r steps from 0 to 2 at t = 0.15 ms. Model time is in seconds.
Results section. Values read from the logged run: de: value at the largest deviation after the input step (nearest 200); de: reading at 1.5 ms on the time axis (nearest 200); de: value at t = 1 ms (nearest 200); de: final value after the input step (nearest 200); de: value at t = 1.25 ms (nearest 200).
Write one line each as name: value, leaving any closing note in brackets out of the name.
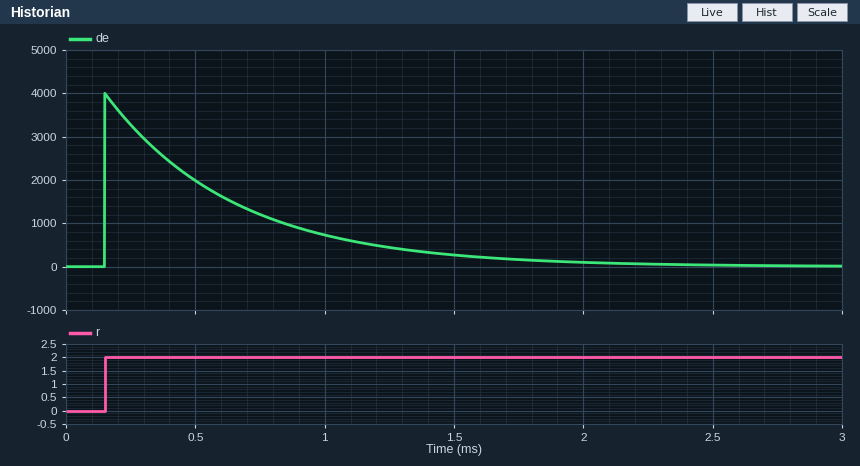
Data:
de: value at the largest deviation after the input step: 4000
de: reading at 1.5 ms on the time axis: 200
de: value at t = 1 ms: 800
de: final value after the input step: 0
de: value at t = 1.25 ms: 400
